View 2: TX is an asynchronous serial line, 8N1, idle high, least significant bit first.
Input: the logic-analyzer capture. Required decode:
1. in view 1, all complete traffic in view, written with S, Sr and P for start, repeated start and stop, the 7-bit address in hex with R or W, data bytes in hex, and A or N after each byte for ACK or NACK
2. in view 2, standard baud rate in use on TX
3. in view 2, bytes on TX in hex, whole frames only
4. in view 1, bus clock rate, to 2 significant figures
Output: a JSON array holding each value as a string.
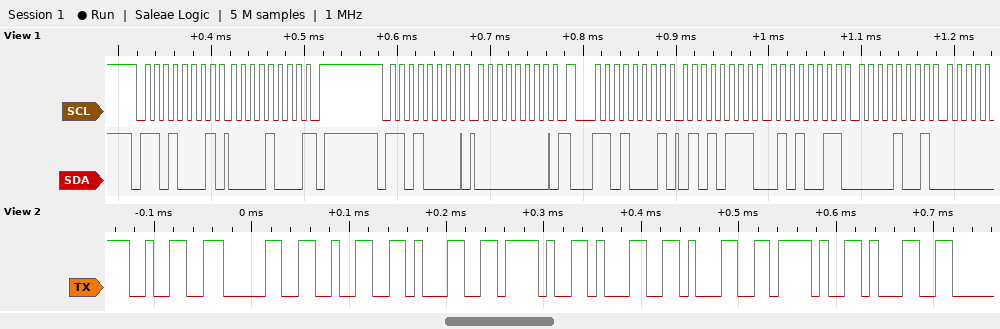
["S 68R A 08 N P S 68W A 00 A Sr 68R A 57 A 53 A 09 A", "115200 baud", "32 30 32 31 2F 31 31 2F 31", "100 kHz"]
